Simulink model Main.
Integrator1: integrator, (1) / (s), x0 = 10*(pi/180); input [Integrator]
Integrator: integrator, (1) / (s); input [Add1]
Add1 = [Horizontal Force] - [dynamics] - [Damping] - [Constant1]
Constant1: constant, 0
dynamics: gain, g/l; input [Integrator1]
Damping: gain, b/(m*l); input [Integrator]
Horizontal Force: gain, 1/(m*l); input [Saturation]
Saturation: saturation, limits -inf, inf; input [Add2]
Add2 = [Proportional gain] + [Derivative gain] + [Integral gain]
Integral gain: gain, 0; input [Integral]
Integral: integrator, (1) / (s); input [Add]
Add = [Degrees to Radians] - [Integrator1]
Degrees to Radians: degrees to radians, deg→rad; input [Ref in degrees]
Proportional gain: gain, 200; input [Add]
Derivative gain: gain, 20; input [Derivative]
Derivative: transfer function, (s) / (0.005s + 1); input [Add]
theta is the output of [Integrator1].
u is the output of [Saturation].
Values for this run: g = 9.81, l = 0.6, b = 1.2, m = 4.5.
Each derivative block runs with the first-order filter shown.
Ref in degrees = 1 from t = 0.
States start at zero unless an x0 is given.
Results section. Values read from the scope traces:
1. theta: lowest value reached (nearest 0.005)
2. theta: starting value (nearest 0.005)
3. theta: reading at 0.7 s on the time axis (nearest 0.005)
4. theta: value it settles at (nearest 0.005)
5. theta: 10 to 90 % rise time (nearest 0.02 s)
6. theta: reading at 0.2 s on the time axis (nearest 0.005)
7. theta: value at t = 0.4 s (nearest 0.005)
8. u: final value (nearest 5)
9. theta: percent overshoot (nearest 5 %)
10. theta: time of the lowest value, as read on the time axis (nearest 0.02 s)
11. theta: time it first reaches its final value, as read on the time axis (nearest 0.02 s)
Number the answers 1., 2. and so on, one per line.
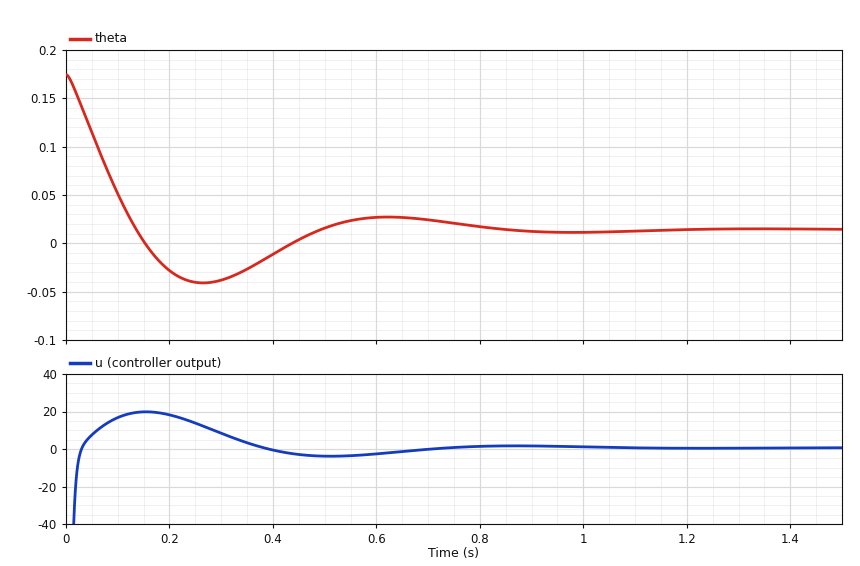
1. -0.040
2. 0.175
3. 0.025
4. 0.015
5. 0.10 s
6. -0.030
7. -0.010
8. 0
9. 35 %
10. 0.26 s
11. 0.14 s
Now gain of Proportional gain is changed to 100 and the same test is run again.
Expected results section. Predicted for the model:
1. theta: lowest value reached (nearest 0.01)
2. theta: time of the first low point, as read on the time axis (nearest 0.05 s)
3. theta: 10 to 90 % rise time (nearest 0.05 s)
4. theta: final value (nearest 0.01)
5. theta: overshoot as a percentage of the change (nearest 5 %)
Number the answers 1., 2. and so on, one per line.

1. -0.03
2. 0.35 s
3. 0.15 s
4. 0.01
5. 25 %
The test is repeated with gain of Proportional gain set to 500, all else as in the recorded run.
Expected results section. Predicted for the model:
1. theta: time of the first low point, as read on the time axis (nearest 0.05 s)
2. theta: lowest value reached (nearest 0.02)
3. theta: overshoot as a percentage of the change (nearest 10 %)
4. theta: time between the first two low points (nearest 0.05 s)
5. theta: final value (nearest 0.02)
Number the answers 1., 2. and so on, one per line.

1. 0.20 s
2. -0.06
3. 50 %
4. 0.45 s
5. 0.02
